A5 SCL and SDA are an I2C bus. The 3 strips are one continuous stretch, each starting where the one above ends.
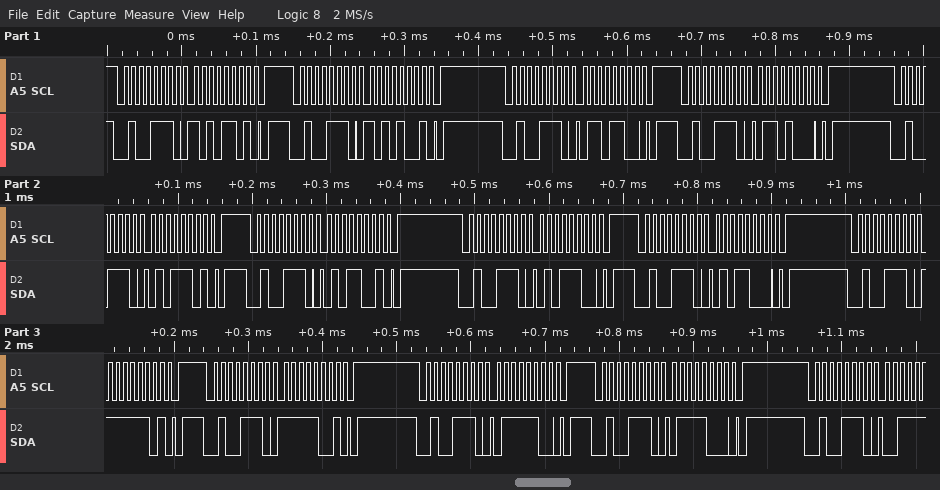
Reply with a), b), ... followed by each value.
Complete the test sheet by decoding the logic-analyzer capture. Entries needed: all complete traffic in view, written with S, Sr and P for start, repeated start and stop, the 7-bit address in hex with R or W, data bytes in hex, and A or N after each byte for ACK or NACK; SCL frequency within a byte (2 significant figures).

a) S 27W A AD A P S 27W A A9 A P S 27W A 6C A P S 27W A 68 A P S 27W A 5D A P S 27W A 59 A P S 27W A 5C A P S 27W A 58 A P S 27W A FD A P S 27W A F9 A P S 27W A 7C A P S 27W A 78 A P S 27W A
b) 100 kHz
